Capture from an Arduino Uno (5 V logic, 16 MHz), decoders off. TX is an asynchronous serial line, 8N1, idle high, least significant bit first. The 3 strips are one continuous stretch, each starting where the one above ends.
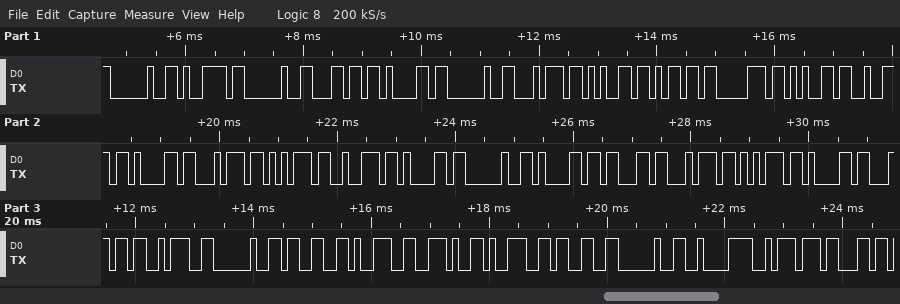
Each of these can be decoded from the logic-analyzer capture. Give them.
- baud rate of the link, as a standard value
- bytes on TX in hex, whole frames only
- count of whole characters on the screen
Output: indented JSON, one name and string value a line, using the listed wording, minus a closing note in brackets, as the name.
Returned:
{
  "baud rate of the link, as a standard value": "9600 baud",
  "bytes on TX in hex, whole frames only": "0x20 0x79 0x20 0x6C 0x61 0x20 0x74 0x65 0x6D 0x70 0x65 0x72 0x61 0x74 0x75 0x72 0x61 0x20 0x61 0x63 0x74 0x75 0x61 0x6C 0x3A 0x20 0x33 0x39 0x2E 0x39 0x33 0x20 0xC2 0xBA 0x63",
  "count of whole characters on the screen": "35"
}
